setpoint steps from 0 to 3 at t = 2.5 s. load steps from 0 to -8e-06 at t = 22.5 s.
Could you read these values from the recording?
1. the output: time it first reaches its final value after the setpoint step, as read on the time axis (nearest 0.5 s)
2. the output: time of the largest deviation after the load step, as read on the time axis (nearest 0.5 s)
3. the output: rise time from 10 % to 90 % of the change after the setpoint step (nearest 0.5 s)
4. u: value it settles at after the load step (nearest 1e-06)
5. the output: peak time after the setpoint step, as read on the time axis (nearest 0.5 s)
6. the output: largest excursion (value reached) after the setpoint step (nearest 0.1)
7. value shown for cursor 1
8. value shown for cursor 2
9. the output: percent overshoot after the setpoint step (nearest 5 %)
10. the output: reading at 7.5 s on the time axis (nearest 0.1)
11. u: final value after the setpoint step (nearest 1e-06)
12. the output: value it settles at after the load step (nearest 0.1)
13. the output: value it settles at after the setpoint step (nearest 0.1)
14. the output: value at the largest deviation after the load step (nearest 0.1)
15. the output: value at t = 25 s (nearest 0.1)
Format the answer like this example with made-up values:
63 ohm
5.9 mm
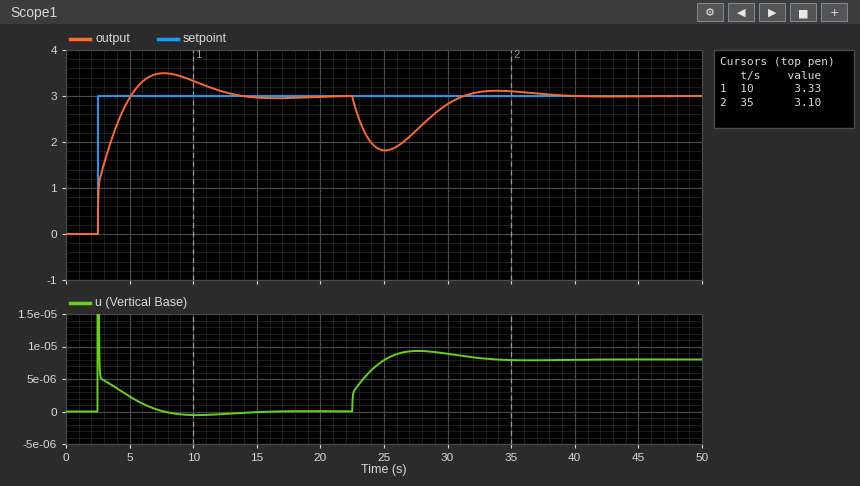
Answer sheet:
5.0 s
25.0 s
2.0 s
0.000008
7.5 s
3.5
3.33
3.10
15 %
3.5
0.000000
3.0
3.0
1.8
1.8
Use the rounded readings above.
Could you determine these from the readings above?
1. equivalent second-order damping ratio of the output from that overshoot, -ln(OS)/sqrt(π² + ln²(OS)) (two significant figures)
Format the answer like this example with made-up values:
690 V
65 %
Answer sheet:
0.52
